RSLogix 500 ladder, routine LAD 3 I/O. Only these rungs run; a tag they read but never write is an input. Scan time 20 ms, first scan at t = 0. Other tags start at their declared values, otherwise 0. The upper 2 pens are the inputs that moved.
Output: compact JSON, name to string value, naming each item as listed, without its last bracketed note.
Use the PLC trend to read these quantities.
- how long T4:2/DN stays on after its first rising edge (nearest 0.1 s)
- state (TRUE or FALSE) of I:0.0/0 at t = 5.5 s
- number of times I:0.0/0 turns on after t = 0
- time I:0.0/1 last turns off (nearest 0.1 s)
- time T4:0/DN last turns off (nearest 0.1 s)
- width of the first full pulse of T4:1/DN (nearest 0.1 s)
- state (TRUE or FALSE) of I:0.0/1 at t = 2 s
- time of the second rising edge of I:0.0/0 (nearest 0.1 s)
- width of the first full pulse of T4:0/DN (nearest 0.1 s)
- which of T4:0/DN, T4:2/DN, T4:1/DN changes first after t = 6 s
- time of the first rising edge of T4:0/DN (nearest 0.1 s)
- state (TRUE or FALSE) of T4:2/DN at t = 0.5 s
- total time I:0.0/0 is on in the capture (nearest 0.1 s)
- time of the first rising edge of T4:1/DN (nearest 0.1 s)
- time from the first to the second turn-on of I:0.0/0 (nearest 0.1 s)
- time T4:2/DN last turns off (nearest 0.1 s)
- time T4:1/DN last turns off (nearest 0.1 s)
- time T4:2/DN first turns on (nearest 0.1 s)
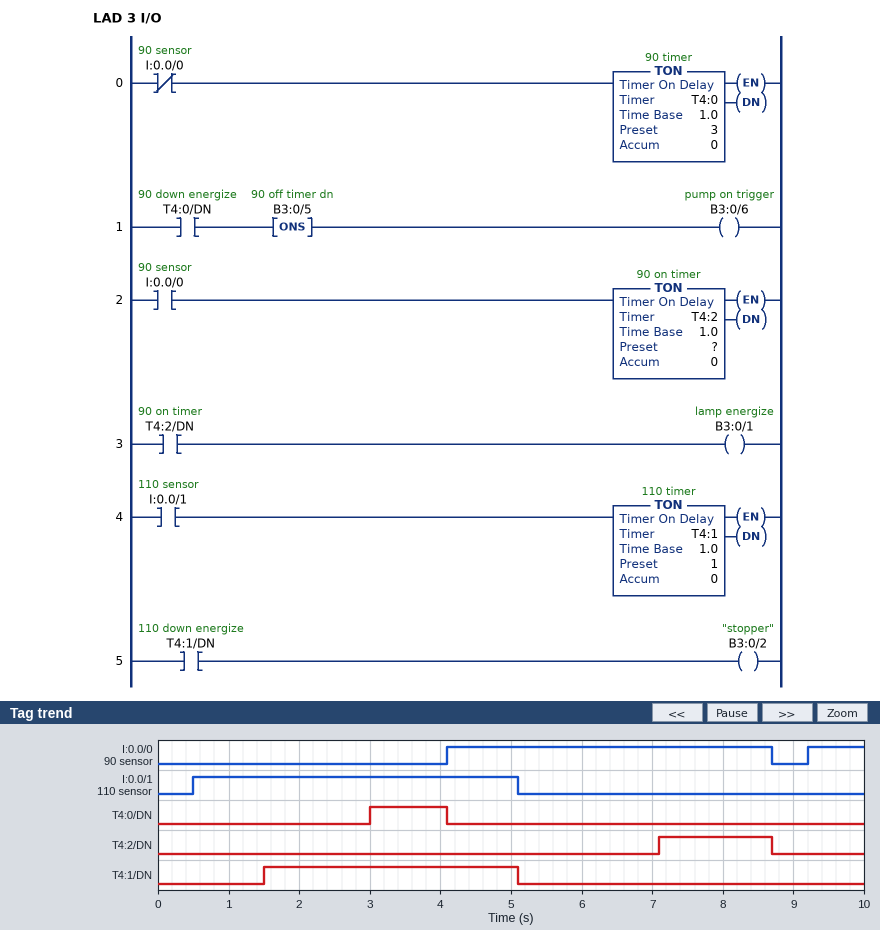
{"how long T4:2/DN stays on after its first rising edge": "1.6 s", "state (TRUE or FALSE) of I:0.0/0 at t = 5.5 s": "TRUE", "number of times I:0.0/0 turns on after t = 0": "2", "time I:0.0/1 last turns off": "5.1 s", "time T4:0/DN last turns off": "4.1 s", "width of the first full pulse of T4:1/DN": "3.6 s", "state (TRUE or FALSE) of I:0.0/1 at t = 2 s": "TRUE", "time of the second rising edge of I:0.0/0": "9.2 s", "width of the first full pulse of T4:0/DN": "1.1 s", "which of T4:0/DN, T4:2/DN, T4:1/DN changes first after t = 6 s": "T4:2/DN", "time of the first rising edge of T4:0/DN": "3.0 s", "state (TRUE or FALSE) of T4:2/DN at t = 0.5 s": "FALSE", "total time I:0.0/0 is on in the capture": "5.4 s", "time of the first rising edge of T4:1/DN": "1.5 s", "time from the first to the second turn-on of I:0.0/0": "5.1 s", "time T4:2/DN last turns off": "8.7 s", "time T4:1/DN last turns off": "5.1 s", "time T4:2/DN first turns on": "7.1 s"}
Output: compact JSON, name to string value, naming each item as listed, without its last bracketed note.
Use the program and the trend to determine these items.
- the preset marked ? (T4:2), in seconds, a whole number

{"the preset marked ? (T4:2), in seconds, a whole number": "3 s"}
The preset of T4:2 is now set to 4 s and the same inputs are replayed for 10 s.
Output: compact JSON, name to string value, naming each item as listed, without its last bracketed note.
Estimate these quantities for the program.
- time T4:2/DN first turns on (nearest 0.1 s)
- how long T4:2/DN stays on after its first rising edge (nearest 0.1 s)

{"time T4:2/DN first turns on": "8.1 s", "how long T4:2/DN stays on after its first rising edge": "0.6 s"}
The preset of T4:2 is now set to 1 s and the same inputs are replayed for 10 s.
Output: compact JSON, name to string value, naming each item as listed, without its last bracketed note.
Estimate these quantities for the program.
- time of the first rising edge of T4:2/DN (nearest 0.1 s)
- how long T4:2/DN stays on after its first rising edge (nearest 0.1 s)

{"time of the first rising edge of T4:2/DN": "5.1 s", "how long T4:2/DN stays on after its first rising edge": "3.6 s"}
